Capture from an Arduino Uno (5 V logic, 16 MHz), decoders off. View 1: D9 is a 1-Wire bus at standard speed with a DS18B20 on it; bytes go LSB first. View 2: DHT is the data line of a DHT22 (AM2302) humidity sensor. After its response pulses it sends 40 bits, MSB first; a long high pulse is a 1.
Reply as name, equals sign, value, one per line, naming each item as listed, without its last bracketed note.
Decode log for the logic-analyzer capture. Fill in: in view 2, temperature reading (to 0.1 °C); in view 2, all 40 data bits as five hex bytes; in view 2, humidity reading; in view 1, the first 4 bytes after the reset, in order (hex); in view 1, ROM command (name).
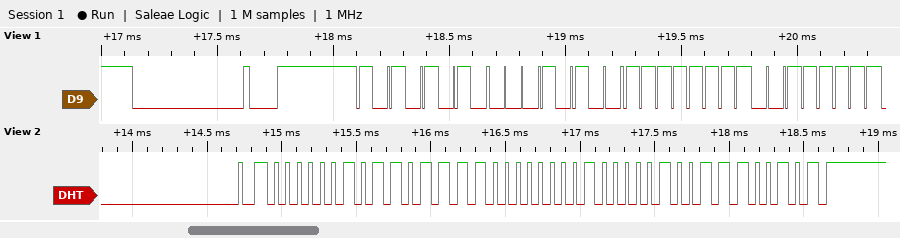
in view 2, temperature reading = 26.0 °C
in view 2, all 40 data bits as five hex bytes = 02 DE 01 04 E5
in view 2, humidity reading = 73.4 %
in view 1, the first 4 bytes after the reset, in order = 55 28 FF FC
in view 1, ROM command = Match ROM
